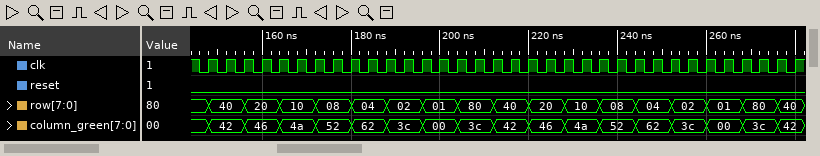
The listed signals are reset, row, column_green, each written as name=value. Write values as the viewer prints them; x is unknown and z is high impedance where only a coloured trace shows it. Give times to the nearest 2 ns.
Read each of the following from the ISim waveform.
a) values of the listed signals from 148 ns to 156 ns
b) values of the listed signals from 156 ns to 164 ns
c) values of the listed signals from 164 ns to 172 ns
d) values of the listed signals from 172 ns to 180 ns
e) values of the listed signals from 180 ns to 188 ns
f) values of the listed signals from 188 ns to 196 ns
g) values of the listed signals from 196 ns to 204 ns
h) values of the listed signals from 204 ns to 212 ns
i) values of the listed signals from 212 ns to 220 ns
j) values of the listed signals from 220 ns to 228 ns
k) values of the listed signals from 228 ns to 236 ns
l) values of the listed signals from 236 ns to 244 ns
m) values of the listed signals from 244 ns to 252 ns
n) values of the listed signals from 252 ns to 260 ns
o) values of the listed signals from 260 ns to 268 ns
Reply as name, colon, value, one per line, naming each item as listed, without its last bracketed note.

values of the listed signals from 148 ns to 156 ns: reset=0, row=40, column_green=42
values of the listed signals from 156 ns to 164 ns: reset=0, row=20, column_green=46
values of the listed signals from 164 ns to 172 ns: reset=0, row=10, column_green=4a
values of the listed signals from 172 ns to 180 ns: reset=0, row=08, column_green=52
values of the listed signals from 180 ns to 188 ns: reset=0, row=04, column_green=62
values of the listed signals from 188 ns to 196 ns: reset=0, row=02, column_green=3c
values of the listed signals from 196 ns to 204 ns: reset=0, row=01, column_green=00
values of the listed signals from 204 ns to 212 ns: reset=0, row=80, column_green=3c
values of the listed signals from 212 ns to 220 ns: reset=0, row=40, column_green=42
values of the listed signals from 220 ns to 228 ns: reset=0, row=20, column_green=46
values of the listed signals from 228 ns to 236 ns: reset=0, row=10, column_green=4a
values of the listed signals from 236 ns to 244 ns: reset=0, row=08, column_green=52
values of the listed signals from 244 ns to 252 ns: reset=0, row=04, column_green=62
values of the listed signals from 252 ns to 260 ns: reset=0, row=02, column_green=3c
values of the listed signals from 260 ns to 268 ns: reset=0, row=01, column_green=00
